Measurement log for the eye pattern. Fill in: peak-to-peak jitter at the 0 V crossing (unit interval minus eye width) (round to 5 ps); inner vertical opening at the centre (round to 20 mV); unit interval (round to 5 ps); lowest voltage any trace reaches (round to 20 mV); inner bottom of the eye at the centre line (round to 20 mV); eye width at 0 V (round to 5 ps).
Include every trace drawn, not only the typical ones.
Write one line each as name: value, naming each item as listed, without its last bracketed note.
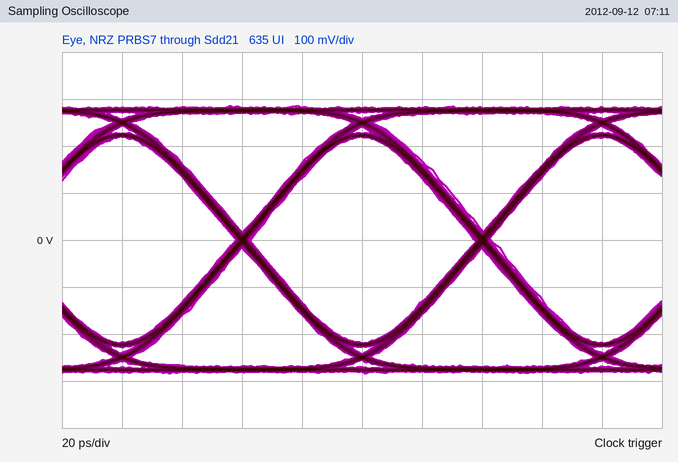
peak-to-peak jitter at the 0 V crossing (unit interval minus eye width): 5 ps
inner vertical opening at the centre: 440 mV
unit interval: 80 ps
lowest voltage any trace reaches: -280 mV
inner bottom of the eye at the centre line: -220 mV
eye width at 0 V: 75 ps
